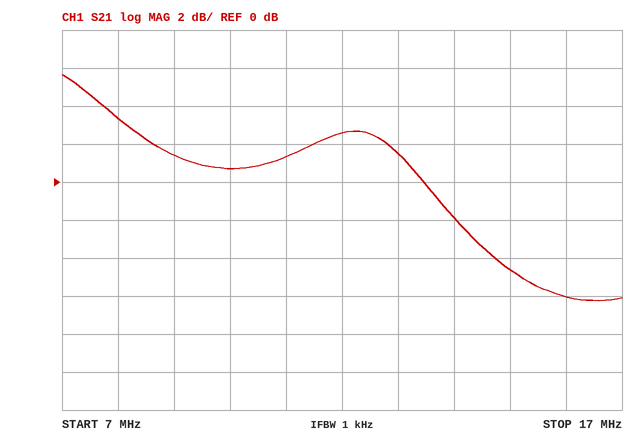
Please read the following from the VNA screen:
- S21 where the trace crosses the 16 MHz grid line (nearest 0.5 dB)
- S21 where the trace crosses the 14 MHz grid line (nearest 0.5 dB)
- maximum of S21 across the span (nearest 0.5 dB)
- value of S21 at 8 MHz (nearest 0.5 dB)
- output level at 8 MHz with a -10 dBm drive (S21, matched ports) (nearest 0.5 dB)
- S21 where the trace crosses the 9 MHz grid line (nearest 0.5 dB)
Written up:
-6.0 dB
-2.0 dB
5.5 dB
3.5 dB
-6.5 dBm
1.5 dB
